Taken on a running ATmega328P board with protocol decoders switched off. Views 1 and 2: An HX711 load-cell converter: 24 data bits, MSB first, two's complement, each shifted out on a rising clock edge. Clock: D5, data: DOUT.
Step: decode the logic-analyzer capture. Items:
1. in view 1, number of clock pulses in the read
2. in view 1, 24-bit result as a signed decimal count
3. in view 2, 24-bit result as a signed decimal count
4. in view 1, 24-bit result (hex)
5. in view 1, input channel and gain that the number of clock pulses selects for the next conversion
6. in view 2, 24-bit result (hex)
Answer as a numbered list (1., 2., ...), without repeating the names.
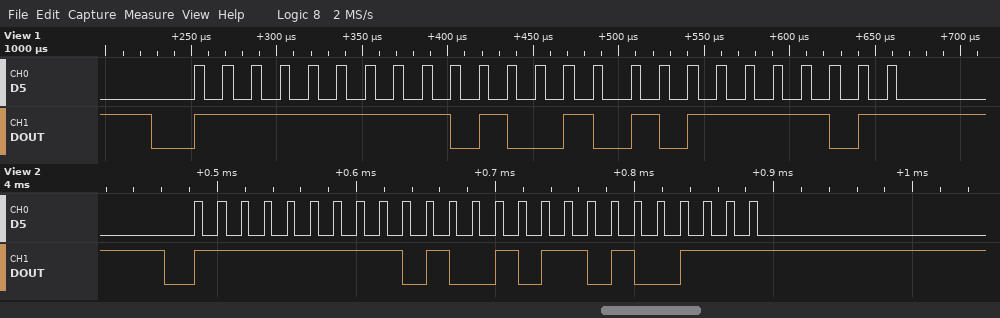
1. 25
2. -23171
3. -23129
4. 0xFFA57D
5. channel A, gain 128
6. 0xFFA5A7
